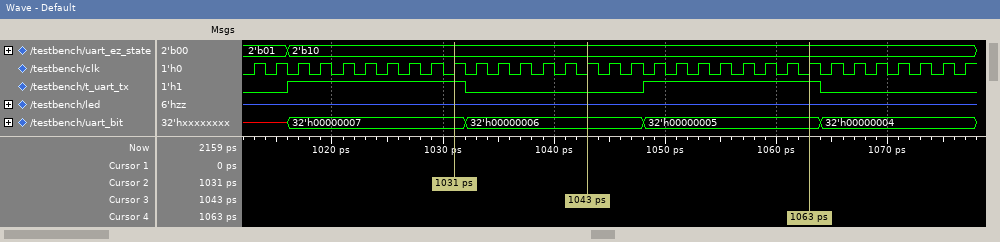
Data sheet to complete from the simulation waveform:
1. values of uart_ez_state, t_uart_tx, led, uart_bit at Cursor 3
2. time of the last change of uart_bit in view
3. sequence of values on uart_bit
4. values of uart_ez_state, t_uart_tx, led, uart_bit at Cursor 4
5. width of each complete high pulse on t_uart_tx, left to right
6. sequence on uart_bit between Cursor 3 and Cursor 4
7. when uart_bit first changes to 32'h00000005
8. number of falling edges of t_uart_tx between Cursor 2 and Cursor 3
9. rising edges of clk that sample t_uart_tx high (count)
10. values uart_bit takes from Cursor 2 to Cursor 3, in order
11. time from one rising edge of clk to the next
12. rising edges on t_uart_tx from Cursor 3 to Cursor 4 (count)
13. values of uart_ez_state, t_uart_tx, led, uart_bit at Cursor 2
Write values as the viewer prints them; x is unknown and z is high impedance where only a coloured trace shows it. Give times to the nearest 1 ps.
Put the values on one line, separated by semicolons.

uart_ez_state=2'b10, t_uart_tx=0, led=z, uart_bit=32'h00000006; 1064 ps; x, 32'h00000007, 32'h00000006, 32'h00000005, 32'h00000004; uart_ez_state=2'b10, t_uart_tx=1, led=z, uart_bit=32'h00000005; 16 ps, 16 ps; 32'h00000006, 32'h00000005; 1048 ps; 1; 16; 32'h00000007, 32'h00000006; 2 ps; 1; uart_ez_state=2'b10, t_uart_tx=1, led=z, uart_bit=32'h00000007
